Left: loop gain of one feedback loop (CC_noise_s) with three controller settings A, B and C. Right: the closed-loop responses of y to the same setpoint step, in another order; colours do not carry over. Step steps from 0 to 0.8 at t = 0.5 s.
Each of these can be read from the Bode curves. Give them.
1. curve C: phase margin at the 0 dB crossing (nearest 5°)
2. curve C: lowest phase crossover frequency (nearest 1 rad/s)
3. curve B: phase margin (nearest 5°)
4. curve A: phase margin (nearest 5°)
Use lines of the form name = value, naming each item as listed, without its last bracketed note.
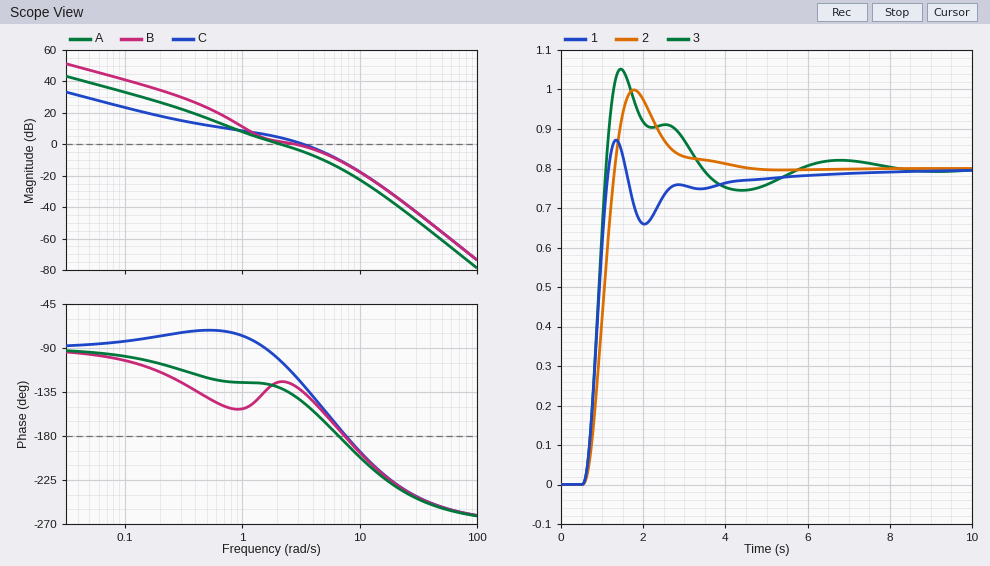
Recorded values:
curve C: phase margin at the 0 dB crossing = 50°
curve C: lowest phase crossover frequency = 8 rad/s
curve B: phase margin = 50°
curve A: phase margin = 50°
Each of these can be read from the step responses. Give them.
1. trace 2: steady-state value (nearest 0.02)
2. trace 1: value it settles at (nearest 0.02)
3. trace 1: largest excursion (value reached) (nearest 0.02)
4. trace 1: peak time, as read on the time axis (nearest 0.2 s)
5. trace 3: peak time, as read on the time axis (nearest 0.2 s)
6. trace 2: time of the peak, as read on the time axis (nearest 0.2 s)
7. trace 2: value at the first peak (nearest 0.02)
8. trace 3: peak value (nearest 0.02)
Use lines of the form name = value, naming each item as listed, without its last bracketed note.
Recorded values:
trace 2: steady-state value = 0.80
trace 1: value it settles at = 0.80
trace 1: largest excursion (value reached) = 0.88
trace 1: peak time, as read on the time axis = 1.4 s
trace 3: peak time, as read on the time axis = 1.4 s
trace 2: time of the peak, as read on the time axis = 1.8 s
trace 2: value at the first peak = 1.00
trace 3: peak value = 1.06
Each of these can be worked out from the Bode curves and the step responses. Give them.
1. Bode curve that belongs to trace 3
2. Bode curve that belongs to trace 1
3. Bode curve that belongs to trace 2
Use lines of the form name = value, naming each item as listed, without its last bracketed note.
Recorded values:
Bode curve that belongs to trace 3 = B
Bode curve that belongs to trace 1 = C
Bode curve that belongs to trace 2 = A
